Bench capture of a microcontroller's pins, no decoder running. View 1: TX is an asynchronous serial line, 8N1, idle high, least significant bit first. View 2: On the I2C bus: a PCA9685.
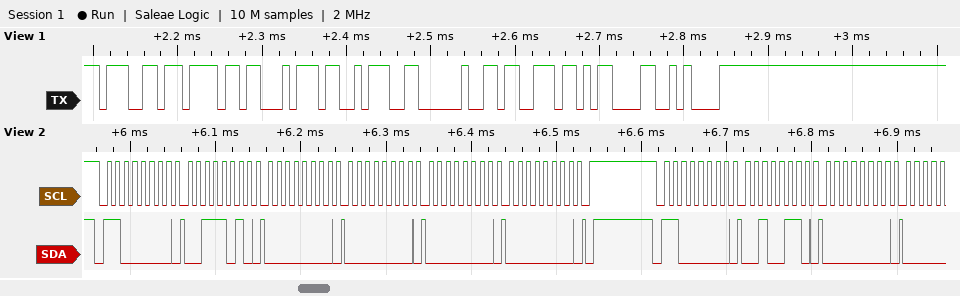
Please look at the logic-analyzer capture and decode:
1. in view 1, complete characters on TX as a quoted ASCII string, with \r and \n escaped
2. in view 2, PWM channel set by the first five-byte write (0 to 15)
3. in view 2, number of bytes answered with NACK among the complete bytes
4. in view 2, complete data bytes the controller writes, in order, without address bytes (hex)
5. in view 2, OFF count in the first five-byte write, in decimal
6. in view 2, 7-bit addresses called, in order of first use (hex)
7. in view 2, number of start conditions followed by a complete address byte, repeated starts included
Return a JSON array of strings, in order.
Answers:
["\"got: s\\r\\n\"", "13", "0", "3A 00 00 00 00 26 00", "0", "0x60", "2"]
